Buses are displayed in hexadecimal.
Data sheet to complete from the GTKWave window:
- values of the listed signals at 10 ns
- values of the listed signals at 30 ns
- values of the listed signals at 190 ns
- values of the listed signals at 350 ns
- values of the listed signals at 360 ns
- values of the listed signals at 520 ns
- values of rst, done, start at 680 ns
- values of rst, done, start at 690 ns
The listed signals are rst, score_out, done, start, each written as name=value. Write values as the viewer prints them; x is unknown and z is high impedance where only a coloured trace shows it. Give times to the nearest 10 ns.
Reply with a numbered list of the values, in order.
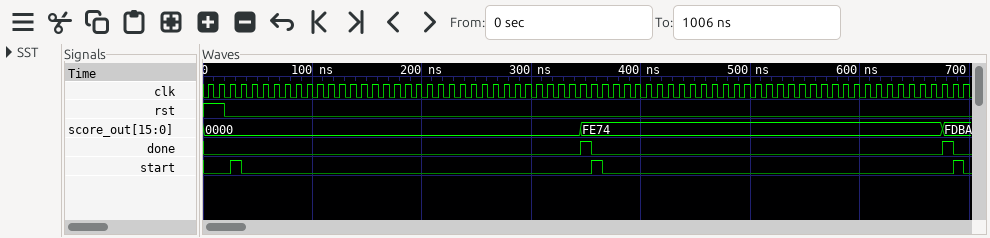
1. rst=1, score_out=0000, done=0, start=0
2. rst=0, score_out=0000, done=0, start=1
3. rst=0, score_out=0000, done=0, start=0
4. rst=0, score_out=FE74, done=1, start=0
5. rst=0, score_out=FE74, done=0, start=1
6. rst=0, score_out=FE74, done=0, start=0
7. rst=0, done=1, start=0
8. rst=0, done=0, start=1
